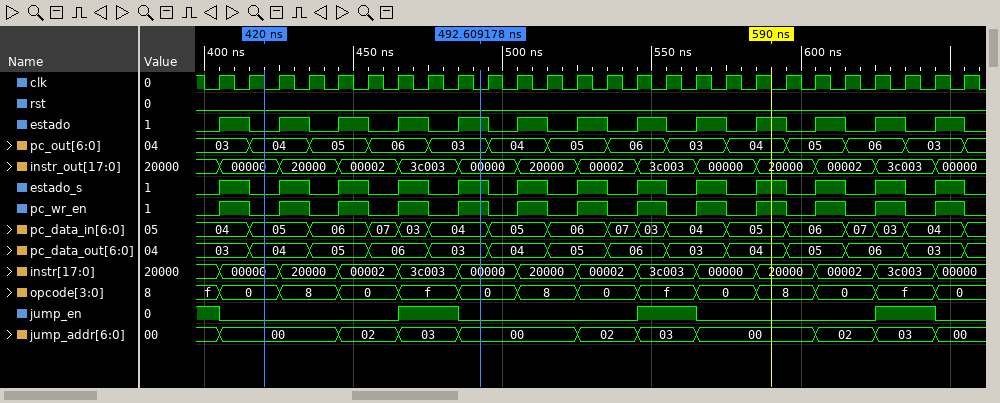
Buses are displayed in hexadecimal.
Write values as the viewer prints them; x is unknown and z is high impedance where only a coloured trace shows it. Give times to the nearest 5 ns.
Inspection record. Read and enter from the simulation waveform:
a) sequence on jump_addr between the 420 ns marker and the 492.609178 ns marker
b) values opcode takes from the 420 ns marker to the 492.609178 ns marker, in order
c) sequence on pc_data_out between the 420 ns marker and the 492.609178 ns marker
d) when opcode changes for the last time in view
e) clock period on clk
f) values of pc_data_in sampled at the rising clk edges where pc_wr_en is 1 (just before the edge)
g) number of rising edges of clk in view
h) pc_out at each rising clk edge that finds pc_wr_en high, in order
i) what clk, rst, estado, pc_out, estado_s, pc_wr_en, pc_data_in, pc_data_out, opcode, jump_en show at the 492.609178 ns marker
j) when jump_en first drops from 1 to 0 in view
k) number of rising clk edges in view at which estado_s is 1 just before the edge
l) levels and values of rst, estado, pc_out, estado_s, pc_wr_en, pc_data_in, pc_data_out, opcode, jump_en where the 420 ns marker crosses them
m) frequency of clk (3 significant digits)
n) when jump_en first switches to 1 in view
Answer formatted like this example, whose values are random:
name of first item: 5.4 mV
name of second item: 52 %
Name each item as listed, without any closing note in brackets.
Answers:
sequence on jump_addr between the 420 ns marker and the 492.609178 ns marker: 00, 02, 03, 00
values opcode takes from the 420 ns marker to the 492.609178 ns marker, in order: 0, 8, 0, f, 0
sequence on pc_data_out between the 420 ns marker and the 492.609178 ns marker: 04, 05, 06, 03
when opcode changes for the last time in view: 645 ns
clock period on clk: 10 ns
values of pc_data_in sampled at the rising clk edges where pc_wr_en is 1: 04, 05, 06, 03, 04, 05, 06, 03, 04, 05, 06, 03, 04
number of rising edges of clk in view: 26
pc_out at each rising clk edge that finds pc_wr_en high, in order: 03, 04, 05, 06, 03, 04, 05, 06, 03, 04, 05, 06, 03
what clk, rst, estado, pc_out, estado_s, pc_wr_en, pc_data_in, pc_data_out, opcode, jump_en show at the 492.609178 ns marker: clk=0, rst=0, estado=1, pc_out=03, estado_s=1, pc_wr_en=1, pc_data_in=04, pc_data_out=03, opcode=0, jump_en=0
when jump_en first drops from 1 to 0 in view: 405 ns
number of rising clk edges in view at which estado_s is 1 just before the edge: 13
levels and values of rst, estado, pc_out, estado_s, pc_wr_en, pc_data_in, pc_data_out, opcode, jump_en where the 420 ns marker crosses them: rst=0, estado=0, pc_out=04, estado_s=0, pc_wr_en=0, pc_data_in=05, pc_data_out=04, opcode=0, jump_en=0
frequency of clk: 100 MHz
when jump_en first switches to 1 in view: 465 ns
